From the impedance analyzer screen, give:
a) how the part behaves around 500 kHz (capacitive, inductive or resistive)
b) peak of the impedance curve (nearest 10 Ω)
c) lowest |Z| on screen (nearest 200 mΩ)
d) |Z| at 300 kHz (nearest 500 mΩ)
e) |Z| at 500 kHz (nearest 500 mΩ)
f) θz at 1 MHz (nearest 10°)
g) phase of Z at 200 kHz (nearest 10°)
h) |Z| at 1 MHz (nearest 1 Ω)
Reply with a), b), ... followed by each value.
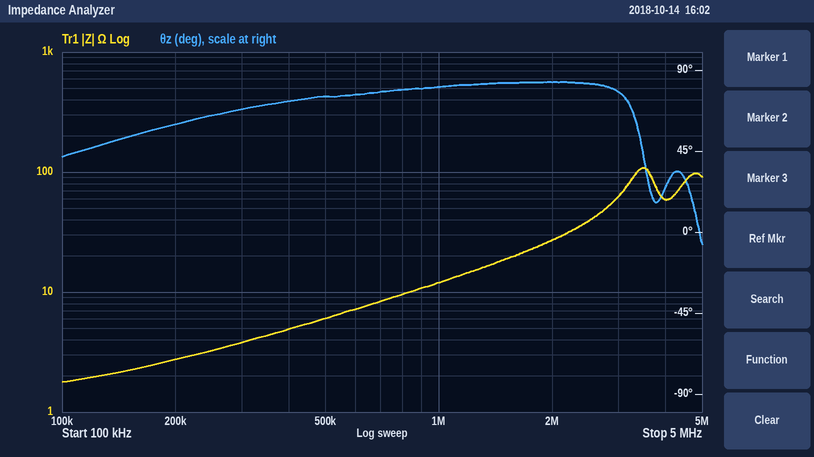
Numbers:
a) inductive
b) 110 Ω
c) 1.8 Ω
d) 4.0 Ω
e) 6.0 Ω
f) 80°
g) 60°
h) 12 Ω
